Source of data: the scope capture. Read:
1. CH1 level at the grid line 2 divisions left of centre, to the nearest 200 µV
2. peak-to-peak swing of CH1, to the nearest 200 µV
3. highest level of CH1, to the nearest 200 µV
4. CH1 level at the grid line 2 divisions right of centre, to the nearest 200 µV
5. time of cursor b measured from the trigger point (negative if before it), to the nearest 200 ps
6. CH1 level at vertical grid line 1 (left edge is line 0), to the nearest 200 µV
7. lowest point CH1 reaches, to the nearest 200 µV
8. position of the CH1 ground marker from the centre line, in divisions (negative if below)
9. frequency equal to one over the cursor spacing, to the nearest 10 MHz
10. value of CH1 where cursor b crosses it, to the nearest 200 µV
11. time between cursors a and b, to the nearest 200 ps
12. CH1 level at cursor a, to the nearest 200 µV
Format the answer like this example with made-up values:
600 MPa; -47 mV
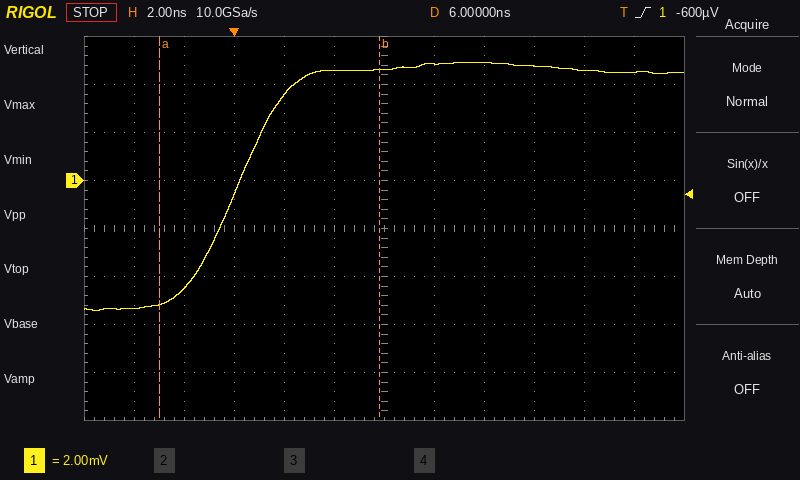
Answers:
3.6 mV; 10.4 mV; 5.0 mV; 5.0 mV; +5.8 ns; -5.4 mV; -5.4 mV; +1.0 div; 110 MHz; 4.6 mV; 8.8 ns; -5.2 mV
